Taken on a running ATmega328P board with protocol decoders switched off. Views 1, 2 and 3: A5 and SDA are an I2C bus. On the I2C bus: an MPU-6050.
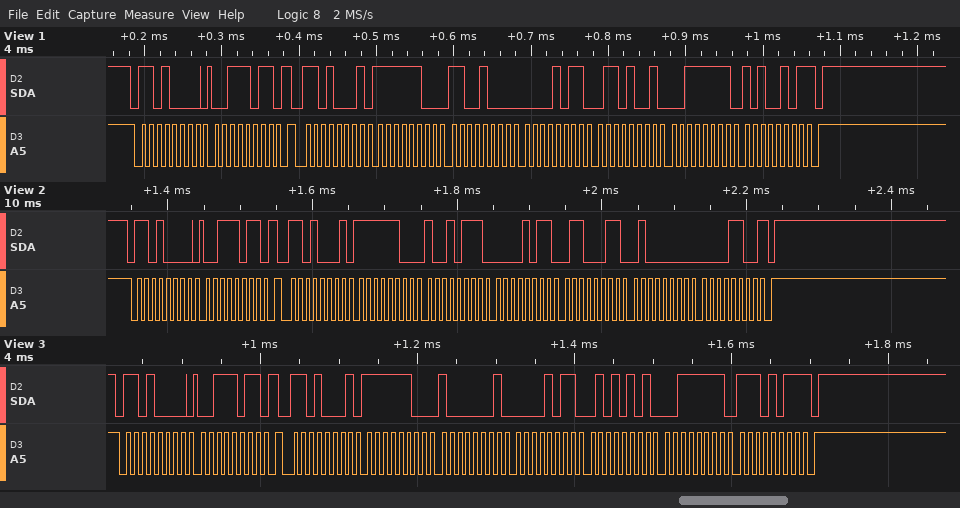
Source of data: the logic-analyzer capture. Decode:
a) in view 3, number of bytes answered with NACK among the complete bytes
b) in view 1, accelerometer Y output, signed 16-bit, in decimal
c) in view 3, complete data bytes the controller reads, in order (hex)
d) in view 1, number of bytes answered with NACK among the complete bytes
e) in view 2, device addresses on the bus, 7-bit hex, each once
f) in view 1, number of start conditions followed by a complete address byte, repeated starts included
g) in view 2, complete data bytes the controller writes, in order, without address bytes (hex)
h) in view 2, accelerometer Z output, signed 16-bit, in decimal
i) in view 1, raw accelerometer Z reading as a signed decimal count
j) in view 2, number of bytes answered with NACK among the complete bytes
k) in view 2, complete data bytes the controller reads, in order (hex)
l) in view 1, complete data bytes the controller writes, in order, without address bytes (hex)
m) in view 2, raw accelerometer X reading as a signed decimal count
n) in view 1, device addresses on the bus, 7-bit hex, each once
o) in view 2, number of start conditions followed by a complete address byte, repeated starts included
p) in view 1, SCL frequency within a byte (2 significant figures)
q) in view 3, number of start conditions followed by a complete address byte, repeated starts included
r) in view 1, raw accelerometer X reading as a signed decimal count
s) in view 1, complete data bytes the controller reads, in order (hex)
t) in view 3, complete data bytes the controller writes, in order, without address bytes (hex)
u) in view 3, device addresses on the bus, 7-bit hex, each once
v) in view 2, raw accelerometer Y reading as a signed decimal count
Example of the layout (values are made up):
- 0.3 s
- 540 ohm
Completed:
- 1
- 2921
- FC 81 0B 55 3F EB
- 1
- 0x68
- 2
- 3B
- 16396
- 16293
- 1
- FC 97 0B 63 40 0C
- 3B
- -873
- 0x68
- 2
- 100 kHz
- 2
- -824
- FC C8 0B 69 3F A5
- 3B
- 0x68
- 2915
